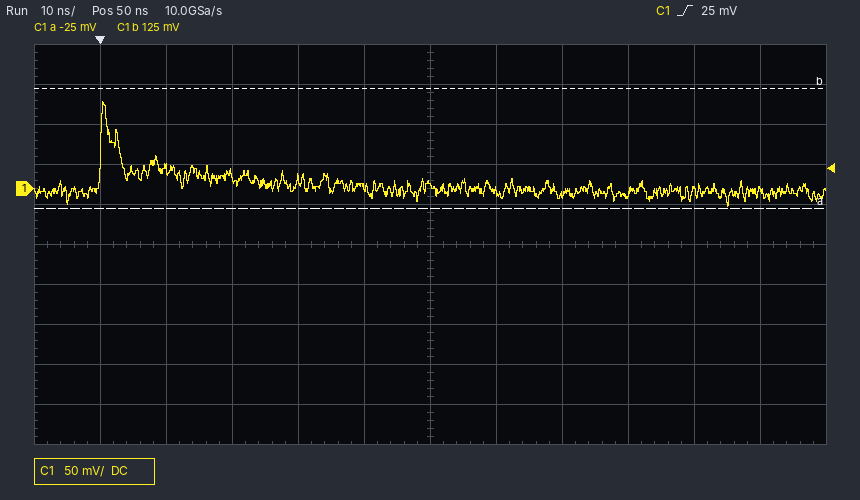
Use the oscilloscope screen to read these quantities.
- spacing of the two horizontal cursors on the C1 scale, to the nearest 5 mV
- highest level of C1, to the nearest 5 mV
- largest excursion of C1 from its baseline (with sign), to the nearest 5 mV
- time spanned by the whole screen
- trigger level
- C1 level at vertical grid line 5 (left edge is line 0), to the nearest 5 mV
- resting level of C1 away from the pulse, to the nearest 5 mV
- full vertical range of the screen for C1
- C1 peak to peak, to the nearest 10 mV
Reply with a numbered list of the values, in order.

1. 150 mV
2. 110 mV
3. +110 mV
4. 120 ns
5. 25 mV
6. 0 mV
7. 0 mV
8. 500 mV
9. 130 mV
